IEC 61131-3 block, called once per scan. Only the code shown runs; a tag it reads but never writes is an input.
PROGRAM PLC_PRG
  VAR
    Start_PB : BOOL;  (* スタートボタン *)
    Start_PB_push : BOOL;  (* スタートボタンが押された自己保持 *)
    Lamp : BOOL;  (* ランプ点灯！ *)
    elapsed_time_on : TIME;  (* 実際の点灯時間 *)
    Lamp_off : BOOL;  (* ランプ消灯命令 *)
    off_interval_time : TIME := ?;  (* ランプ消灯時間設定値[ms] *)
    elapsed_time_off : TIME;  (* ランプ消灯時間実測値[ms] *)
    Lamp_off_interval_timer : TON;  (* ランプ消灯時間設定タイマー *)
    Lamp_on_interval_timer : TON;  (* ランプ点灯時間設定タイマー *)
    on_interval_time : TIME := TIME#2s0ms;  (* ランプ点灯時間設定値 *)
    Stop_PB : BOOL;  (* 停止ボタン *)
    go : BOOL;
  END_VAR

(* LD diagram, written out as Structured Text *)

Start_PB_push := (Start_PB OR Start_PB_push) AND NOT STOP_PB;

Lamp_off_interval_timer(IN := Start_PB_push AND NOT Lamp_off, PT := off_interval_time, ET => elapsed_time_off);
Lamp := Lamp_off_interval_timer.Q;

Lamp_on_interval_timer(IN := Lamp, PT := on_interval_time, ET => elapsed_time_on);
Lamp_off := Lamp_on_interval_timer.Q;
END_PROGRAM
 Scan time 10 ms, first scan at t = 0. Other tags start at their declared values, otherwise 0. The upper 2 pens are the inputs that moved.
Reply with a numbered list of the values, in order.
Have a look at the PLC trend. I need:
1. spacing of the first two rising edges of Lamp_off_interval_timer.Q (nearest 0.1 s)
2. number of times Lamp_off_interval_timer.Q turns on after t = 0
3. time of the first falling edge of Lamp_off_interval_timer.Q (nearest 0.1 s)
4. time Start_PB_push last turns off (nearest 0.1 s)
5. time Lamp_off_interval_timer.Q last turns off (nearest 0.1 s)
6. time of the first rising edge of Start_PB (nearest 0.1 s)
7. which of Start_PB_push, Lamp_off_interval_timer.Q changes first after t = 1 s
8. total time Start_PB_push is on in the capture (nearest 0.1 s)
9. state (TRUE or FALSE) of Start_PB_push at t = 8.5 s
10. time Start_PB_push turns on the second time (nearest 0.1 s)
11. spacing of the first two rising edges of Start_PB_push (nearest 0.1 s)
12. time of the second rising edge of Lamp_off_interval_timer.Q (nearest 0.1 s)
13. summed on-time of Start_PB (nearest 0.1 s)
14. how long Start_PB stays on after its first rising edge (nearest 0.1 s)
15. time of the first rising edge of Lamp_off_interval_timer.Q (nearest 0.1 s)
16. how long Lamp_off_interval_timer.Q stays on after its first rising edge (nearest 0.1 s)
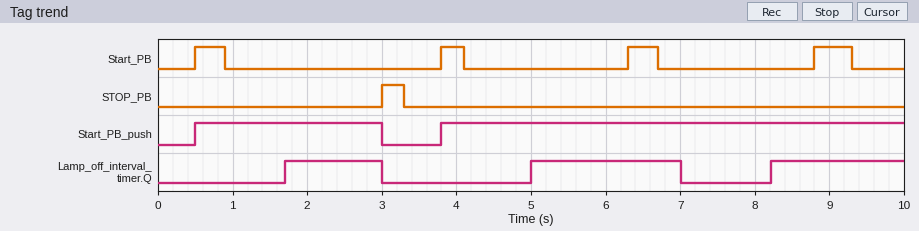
1. 3.3 s
2. 3
3. 3.0 s
4. 3.0 s
5. 7.0 s
6. 0.5 s
7. Lamp_off_interval_timer.Q
8. 8.7 s
9. TRUE
10. 3.8 s
11. 3.3 s
12. 5.0 s
13. 1.6 s
14. 0.4 s
15. 1.7 s
16. 1.3 s
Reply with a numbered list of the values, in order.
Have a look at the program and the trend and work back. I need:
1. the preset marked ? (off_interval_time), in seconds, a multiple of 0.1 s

1. 1.2 s
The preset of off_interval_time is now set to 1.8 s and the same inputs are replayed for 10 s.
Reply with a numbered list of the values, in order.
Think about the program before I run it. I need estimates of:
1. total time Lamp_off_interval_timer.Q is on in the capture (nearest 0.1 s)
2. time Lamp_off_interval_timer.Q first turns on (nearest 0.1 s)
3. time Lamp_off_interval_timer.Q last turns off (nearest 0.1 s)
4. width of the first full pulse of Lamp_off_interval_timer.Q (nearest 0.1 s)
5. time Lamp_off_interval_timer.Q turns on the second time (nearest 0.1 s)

1. 3.3 s
2. 2.3 s
3. 7.6 s
4. 0.7 s
5. 5.6 s
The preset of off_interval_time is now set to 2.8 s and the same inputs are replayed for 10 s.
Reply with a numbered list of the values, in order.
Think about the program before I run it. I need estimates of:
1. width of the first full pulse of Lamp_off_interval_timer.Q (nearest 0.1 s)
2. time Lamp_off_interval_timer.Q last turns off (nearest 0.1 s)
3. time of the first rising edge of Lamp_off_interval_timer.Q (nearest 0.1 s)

1. 2.0 s
2. 8.6 s
3. 6.6 s
